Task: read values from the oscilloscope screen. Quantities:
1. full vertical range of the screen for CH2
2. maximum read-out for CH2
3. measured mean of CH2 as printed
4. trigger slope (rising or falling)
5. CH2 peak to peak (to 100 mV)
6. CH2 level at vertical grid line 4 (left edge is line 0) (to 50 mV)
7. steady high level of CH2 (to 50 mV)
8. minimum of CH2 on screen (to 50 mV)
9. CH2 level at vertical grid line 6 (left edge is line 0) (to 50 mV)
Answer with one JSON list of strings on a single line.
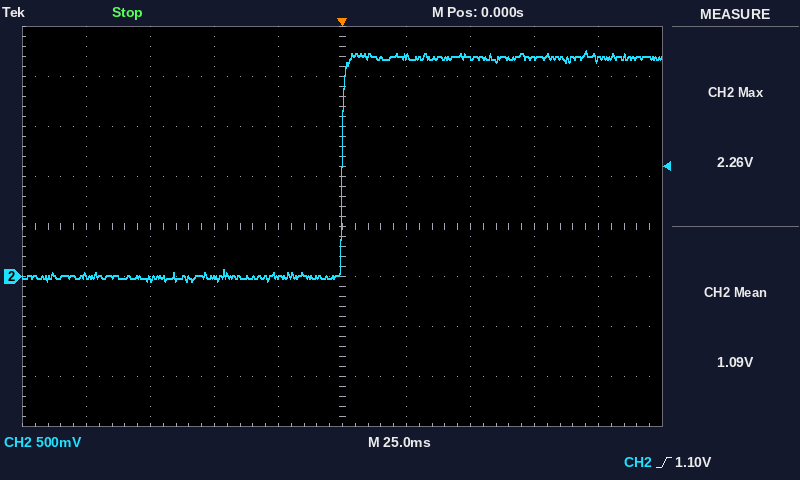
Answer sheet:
["4 V", "2.26 V", "1.09 V", "rising", "2.30 V", "0 mV", "2.20 V", "-50 mV", "2.20 V"]
